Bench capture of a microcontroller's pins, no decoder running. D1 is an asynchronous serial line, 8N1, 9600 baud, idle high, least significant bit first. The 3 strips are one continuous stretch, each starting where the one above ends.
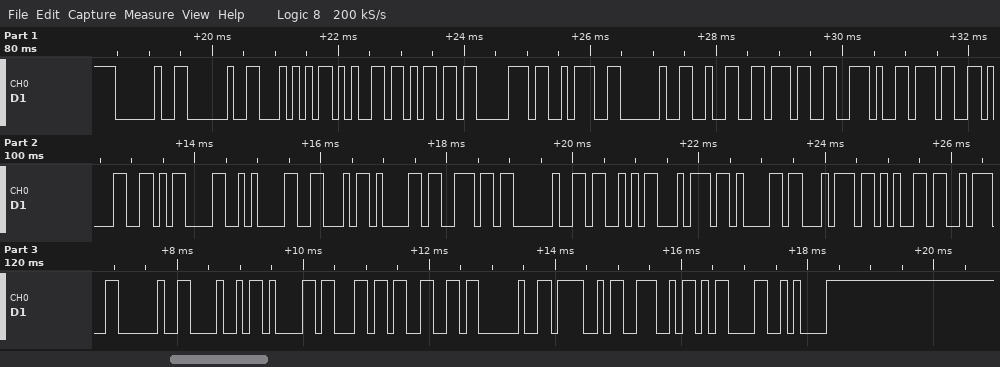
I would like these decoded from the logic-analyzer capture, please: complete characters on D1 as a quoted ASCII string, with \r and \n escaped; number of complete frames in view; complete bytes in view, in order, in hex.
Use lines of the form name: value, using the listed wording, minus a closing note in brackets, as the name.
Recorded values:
complete characters on D1 as a quoted ASCII string, with \r and \n escaped: "  Temp: 27.71\r\nFan State: Half ON\r\n"
number of complete frames in view: 35
complete bytes in view, in order, in hex: 20 20 54 65 6D 70 3A 20 32 37 2E 37 31 0D 0A 46 61 6E 20 53 74 61 74 65 3A 20 48 61 6C 66 20 4F 4E 0D 0A
